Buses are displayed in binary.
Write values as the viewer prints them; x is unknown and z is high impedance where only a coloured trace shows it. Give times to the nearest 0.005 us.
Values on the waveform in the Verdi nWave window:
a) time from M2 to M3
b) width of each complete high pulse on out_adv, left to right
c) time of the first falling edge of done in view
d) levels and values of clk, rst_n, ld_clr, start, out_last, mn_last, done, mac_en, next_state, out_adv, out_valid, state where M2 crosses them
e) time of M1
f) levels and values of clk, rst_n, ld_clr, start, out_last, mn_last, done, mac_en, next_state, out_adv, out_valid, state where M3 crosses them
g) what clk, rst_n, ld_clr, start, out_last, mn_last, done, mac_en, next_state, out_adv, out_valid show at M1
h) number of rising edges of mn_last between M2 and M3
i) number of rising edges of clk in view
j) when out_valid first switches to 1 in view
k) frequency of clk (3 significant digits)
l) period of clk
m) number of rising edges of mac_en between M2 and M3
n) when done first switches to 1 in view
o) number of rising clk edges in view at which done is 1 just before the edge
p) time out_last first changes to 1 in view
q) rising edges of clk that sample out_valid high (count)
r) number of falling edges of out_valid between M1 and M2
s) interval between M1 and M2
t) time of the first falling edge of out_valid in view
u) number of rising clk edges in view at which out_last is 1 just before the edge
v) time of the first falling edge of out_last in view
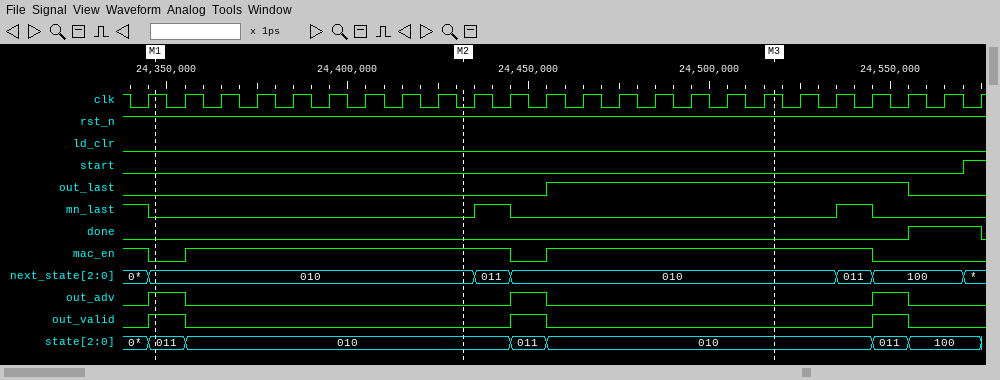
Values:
0.085 us
0.01 us, 0.01 us, 0.01 us
24.575 us
clk=0, rst_n=1, ld_clr=0, start=0, out_last=0, mn_last=0, done=0, mac_en=1, next_state=010, out_adv=0, out_valid=0, state=010
24.345 us
clk=1, rst_n=1, ld_clr=0, start=0, out_last=1, mn_last=0, done=0, mac_en=1, next_state=010, out_adv=0, out_valid=0, state=010
clk=1, rst_n=1, ld_clr=0, start=0, out_last=0, mn_last=0, done=0, mac_en=0, next_state=010, out_adv=1, out_valid=1
1
24
24.345 us
100 MHz
0.01 us
1
24.555 us
2
24.455 us
3
1
0.085 us
24.355 us
10
24.555 us
